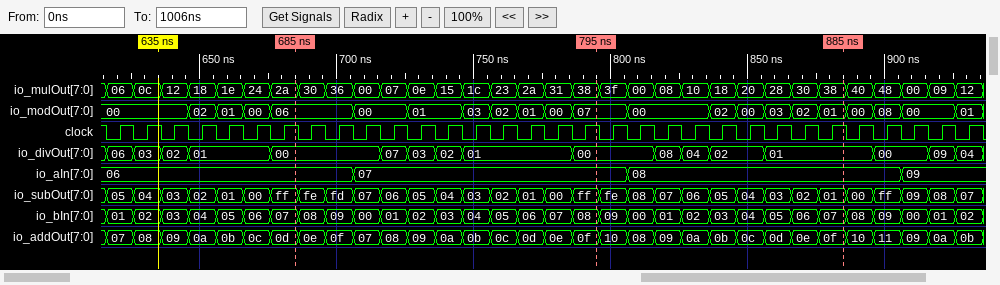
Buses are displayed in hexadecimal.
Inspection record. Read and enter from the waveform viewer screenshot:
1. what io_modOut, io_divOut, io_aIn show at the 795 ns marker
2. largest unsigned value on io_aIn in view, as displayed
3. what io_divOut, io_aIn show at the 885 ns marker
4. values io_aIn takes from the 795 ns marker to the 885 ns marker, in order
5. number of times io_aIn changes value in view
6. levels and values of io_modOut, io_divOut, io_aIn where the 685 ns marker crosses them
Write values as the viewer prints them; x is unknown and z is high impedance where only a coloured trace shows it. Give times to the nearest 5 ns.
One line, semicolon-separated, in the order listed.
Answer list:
io_modOut=07, io_divOut=00, io_aIn=07; 09; io_divOut=01, io_aIn=08; 07, 08; 3; io_modOut=06, io_divOut=00, io_aIn=06
